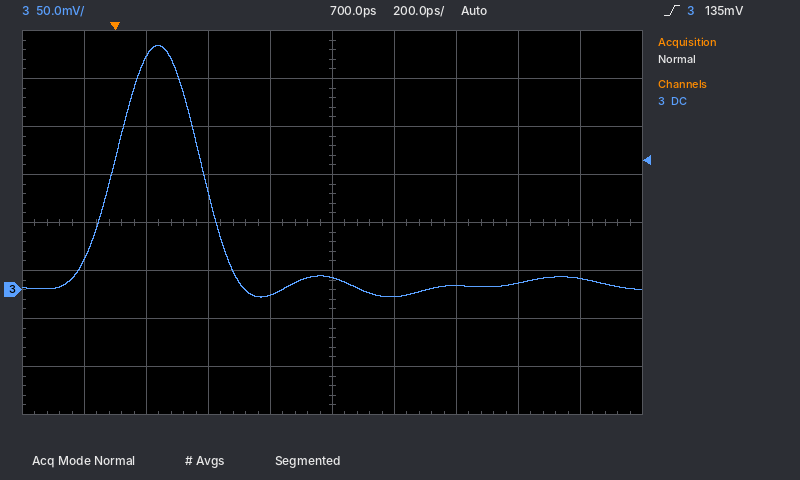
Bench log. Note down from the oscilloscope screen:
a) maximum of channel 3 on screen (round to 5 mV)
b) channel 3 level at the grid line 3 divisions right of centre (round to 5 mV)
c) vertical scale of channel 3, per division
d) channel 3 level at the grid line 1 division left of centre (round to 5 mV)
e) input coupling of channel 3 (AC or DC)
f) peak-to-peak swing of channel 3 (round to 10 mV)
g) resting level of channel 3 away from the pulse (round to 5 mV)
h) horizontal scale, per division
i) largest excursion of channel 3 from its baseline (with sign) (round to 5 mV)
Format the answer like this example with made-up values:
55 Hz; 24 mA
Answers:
255 mV; 5 mV; 50 mV; -5 mV; DC; 260 mV; 5 mV; 200 ps; +250 mV
